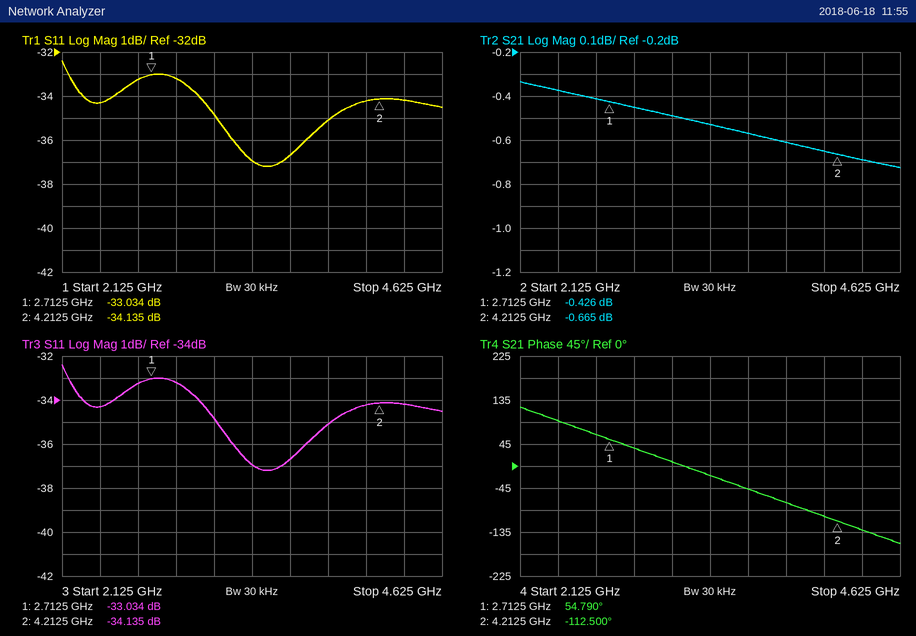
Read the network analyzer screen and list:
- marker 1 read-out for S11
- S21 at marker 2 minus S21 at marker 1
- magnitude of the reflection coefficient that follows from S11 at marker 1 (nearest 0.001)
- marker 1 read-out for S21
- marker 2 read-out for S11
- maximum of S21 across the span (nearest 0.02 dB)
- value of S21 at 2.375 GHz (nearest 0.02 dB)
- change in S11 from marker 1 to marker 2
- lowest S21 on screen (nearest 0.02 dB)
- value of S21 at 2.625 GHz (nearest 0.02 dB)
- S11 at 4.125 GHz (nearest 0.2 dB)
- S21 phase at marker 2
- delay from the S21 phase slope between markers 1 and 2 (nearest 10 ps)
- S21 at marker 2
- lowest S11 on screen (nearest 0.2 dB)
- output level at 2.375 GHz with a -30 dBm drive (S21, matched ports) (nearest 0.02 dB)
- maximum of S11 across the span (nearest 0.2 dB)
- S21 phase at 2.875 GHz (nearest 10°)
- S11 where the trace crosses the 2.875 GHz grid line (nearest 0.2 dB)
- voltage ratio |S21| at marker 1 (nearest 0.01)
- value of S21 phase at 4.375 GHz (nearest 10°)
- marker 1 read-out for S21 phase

-33.034 dB
-0.239 dB
0.022
-0.426 dB
-34.135 dB
-0.34 dB
-0.38 dB
-1.101 dB
-0.72 dB
-0.42 dB
-34.2 dB
-112.500°
310 ps
-0.665 dB
-37.2 dB
-30.38 dBm
-32.4 dB
40°
-33.2 dB
0.95
-130°
54.790°
